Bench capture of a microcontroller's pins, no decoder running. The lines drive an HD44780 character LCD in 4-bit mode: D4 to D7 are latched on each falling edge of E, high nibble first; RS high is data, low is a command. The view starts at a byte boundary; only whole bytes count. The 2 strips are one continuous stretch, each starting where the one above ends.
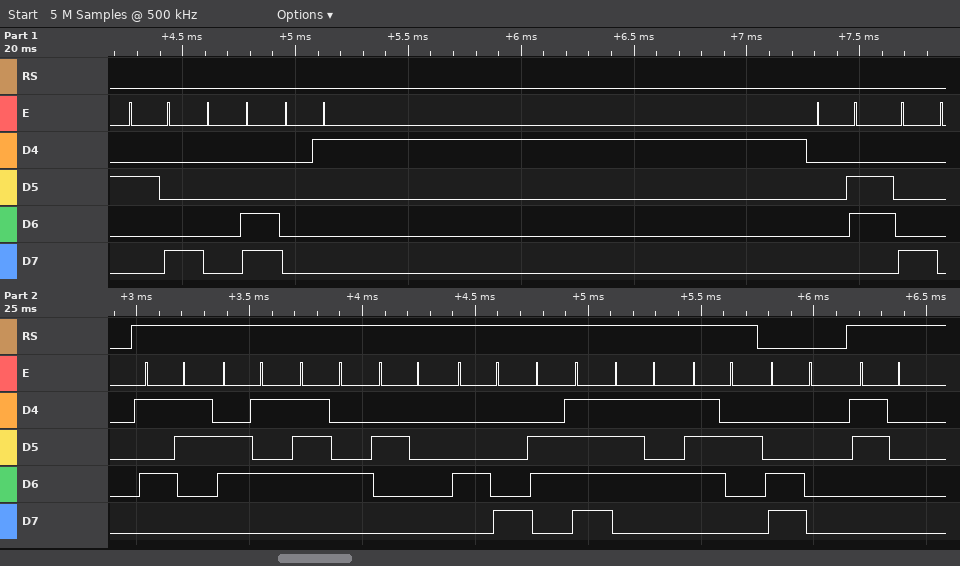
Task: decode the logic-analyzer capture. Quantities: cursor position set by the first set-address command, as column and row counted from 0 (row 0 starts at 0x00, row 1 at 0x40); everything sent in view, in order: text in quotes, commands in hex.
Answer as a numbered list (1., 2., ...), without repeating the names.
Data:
1. column 0, row 0
2. 0x28 0x0C 0x01 0x06 0x80 "Set Hour" 0xC0 "0"
